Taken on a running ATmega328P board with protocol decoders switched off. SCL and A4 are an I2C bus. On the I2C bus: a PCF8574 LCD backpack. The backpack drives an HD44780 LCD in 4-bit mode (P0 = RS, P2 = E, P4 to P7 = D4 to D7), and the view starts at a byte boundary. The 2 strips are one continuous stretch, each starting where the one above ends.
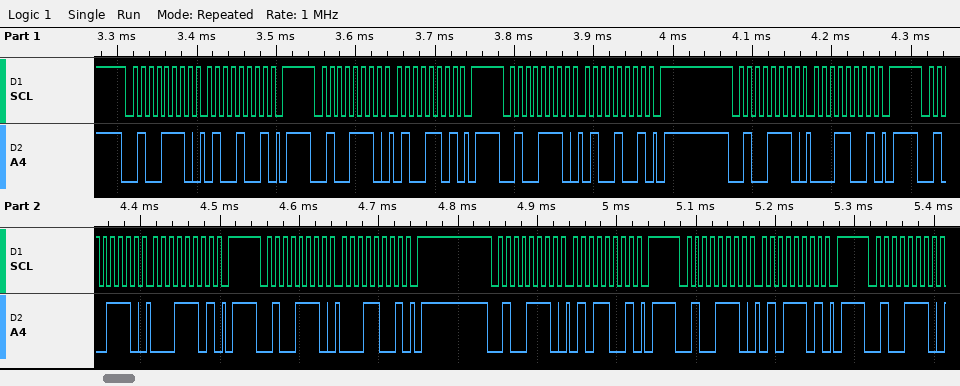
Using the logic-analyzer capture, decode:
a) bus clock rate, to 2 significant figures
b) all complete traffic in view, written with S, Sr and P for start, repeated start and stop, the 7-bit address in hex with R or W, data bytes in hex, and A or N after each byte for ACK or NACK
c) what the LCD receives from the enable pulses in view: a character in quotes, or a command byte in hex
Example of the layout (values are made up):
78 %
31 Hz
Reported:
100 kHz
S 27W A 49 A P S 27W A 4D A P S 27W A 49 A P S 27W A 19 A P S 27W A 1D A P S 27W A 19 A P S 27W A 59 A P S 27W A 5D A P S 27W A
'A'
